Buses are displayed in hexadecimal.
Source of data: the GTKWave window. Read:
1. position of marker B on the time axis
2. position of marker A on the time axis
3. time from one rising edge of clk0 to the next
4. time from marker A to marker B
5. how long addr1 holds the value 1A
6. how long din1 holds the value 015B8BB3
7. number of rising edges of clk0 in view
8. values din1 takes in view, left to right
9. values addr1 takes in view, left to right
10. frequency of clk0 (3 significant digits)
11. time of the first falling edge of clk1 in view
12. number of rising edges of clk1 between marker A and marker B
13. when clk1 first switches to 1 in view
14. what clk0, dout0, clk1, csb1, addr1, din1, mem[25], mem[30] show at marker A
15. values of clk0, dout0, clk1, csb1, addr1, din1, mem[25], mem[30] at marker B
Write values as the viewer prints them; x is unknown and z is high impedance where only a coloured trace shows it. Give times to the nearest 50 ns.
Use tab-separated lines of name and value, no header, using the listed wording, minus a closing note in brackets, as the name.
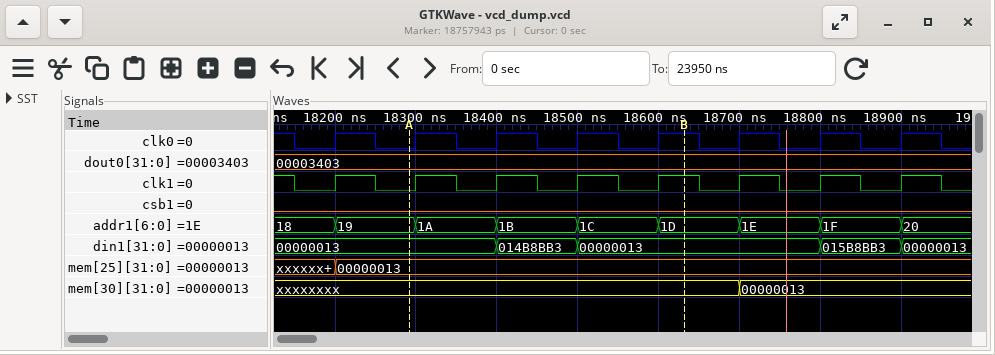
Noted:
position of marker B on the time axis	18650 ns
position of marker A on the time axis	18300 ns
time from one rising edge of clk0 to the next	100 ns
time from marker A to marker B	350 ns
how long addr1 holds the value 1A	100 ns
how long din1 holds the value 015B8BB3	100 ns
number of rising edges of clk0 in view	8
values din1 takes in view, left to right	00000013, 014B8BB3, 00000013, 015B8BB3, 00000013
values addr1 takes in view, left to right	18, 19, 1A, 1B, 1C, 1D, 1E, 1F, 20
frequency of clk0	10.0 MHz
time of the first falling edge of clk1 in view	18150 ns
number of rising edges of clk1 between marker A and marker B	4
when clk1 first switches to 1 in view	18200 ns
what clk0, dout0, clk1, csb1, addr1, din1, mem[25], mem[30] show at marker A	clk0=0, dout0=00003403, clk1=0, csb1=0, addr1=19, din1=00000013, mem[25]=00000013, mem[30]=xxxxxxxx
values of clk0, dout0, clk1, csb1, addr1, din1, mem[25], mem[30] at marker B	clk0=1, dout0=00003403, clk1=1, csb1=0, addr1=1D, din1=00000013, mem[25]=00000013, mem[30]=xxxxxxxx
